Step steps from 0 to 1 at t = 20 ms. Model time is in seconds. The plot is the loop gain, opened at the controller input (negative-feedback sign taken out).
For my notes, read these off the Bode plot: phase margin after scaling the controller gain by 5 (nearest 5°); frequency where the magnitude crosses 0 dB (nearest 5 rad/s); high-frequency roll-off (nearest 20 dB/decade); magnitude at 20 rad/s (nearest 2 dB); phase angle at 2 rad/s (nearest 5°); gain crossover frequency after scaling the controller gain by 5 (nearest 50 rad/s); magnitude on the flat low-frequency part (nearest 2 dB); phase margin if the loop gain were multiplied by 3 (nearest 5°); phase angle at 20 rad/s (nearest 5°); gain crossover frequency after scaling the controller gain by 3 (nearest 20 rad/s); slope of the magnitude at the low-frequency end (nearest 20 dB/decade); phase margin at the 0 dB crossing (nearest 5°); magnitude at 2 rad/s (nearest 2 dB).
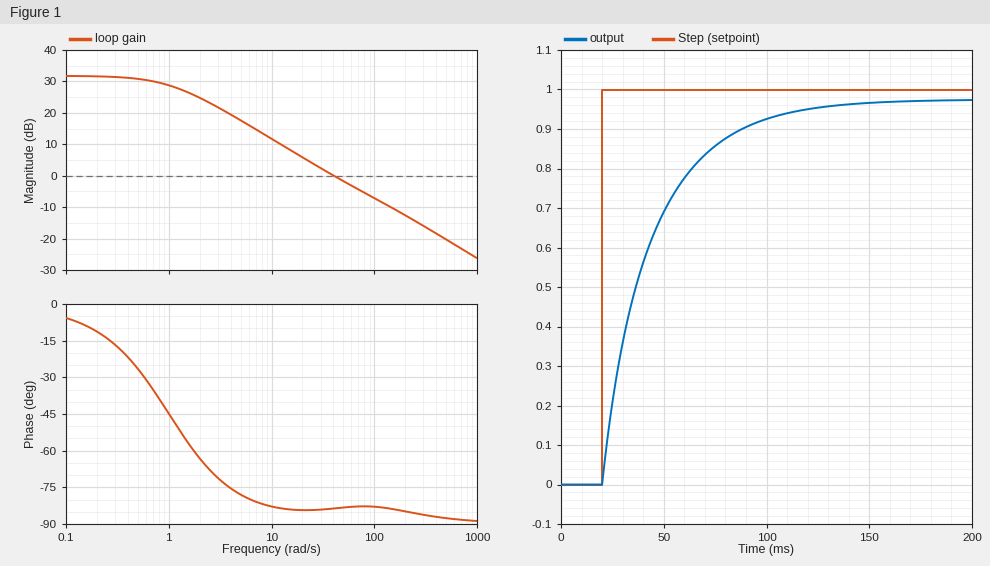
95°
40 rad/s
-20 dB/decade
6 dB
-65°
250 rad/s
32 dB
95°
-85°
140 rad/s
0 dB/decade
95°
24 dB
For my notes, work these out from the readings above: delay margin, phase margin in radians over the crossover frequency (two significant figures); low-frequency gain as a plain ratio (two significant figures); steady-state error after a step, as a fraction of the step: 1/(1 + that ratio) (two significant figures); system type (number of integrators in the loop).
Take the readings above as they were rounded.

0.041 s
40
0.024
0
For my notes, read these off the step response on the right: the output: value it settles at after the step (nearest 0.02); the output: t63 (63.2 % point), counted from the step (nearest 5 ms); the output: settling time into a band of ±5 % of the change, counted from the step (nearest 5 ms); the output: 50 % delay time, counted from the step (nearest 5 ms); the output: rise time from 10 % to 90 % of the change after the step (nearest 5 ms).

0.98
25 ms
80 ms
15 ms
60 ms
